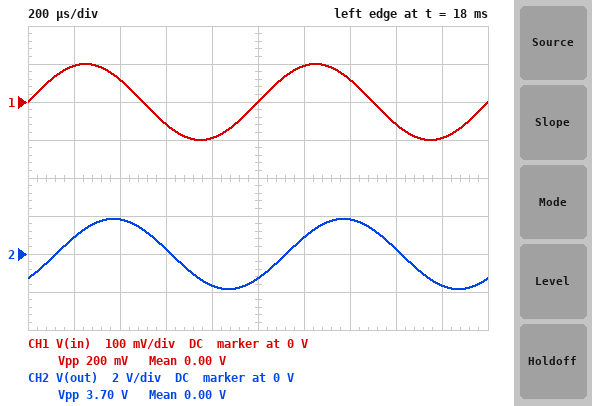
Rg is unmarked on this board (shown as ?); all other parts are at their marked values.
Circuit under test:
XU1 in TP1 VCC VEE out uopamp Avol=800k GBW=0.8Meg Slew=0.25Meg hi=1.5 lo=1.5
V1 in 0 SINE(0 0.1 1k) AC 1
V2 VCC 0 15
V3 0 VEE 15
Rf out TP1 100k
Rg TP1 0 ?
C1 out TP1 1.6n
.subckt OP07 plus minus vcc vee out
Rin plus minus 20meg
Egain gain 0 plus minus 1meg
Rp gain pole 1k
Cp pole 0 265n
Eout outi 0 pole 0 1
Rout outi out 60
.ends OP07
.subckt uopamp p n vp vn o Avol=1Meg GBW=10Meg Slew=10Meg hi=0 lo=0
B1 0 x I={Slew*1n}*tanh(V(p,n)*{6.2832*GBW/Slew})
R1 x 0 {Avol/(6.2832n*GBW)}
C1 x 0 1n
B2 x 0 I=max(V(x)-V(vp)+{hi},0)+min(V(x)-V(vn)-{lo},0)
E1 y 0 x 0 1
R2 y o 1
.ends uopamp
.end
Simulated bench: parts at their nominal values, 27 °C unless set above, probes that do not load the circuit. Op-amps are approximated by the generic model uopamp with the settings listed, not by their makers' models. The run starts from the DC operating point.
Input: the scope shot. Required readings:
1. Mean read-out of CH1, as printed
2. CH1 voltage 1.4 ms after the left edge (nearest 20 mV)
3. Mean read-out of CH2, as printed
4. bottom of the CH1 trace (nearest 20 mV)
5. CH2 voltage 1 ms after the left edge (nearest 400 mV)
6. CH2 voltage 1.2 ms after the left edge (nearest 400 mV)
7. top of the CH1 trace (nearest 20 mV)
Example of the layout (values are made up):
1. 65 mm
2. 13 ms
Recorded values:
1. 0.00 V
2. 60 mV
3. 0.00 V
4. -100 mV
5. -1.2 V
6. 800 mV
7. 100 mV
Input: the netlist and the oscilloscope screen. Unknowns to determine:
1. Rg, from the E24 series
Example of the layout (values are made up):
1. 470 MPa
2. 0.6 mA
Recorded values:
1. 3.9 kΩ
